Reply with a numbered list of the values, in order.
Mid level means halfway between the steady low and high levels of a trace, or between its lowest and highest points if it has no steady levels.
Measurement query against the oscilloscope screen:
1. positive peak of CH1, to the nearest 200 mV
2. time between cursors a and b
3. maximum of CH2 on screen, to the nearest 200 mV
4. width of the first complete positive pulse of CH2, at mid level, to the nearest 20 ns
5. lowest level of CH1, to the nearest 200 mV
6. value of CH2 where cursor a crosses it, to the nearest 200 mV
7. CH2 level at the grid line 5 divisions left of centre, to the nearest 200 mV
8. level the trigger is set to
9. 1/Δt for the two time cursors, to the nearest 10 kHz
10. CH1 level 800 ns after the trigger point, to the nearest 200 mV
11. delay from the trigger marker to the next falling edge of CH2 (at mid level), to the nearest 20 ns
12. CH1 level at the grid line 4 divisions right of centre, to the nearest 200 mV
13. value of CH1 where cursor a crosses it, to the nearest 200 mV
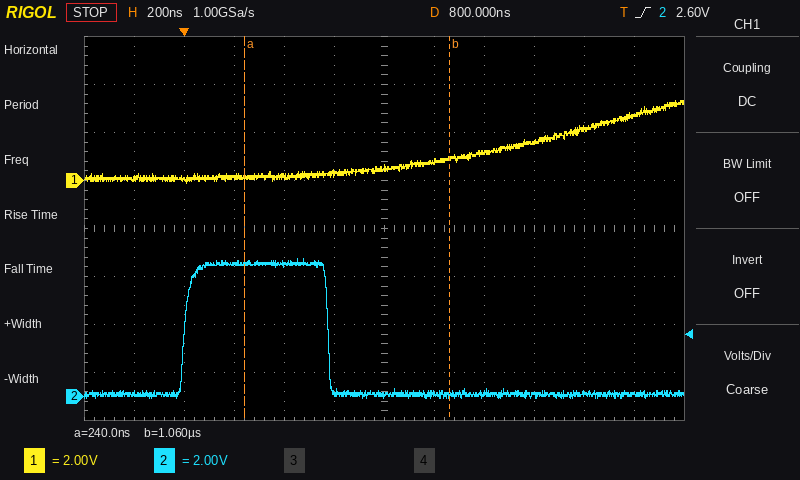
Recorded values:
1. 3.4 V
2. 820 ns
3. 5.8 V
4. 580 ns
5. -200 mV
6. 5.6 V
7. 200 mV
8. 2.60 V
9. 1.22 MHz
10. 600 mV
11. 580 ns
12. 2.2 V
13. 200 mV
